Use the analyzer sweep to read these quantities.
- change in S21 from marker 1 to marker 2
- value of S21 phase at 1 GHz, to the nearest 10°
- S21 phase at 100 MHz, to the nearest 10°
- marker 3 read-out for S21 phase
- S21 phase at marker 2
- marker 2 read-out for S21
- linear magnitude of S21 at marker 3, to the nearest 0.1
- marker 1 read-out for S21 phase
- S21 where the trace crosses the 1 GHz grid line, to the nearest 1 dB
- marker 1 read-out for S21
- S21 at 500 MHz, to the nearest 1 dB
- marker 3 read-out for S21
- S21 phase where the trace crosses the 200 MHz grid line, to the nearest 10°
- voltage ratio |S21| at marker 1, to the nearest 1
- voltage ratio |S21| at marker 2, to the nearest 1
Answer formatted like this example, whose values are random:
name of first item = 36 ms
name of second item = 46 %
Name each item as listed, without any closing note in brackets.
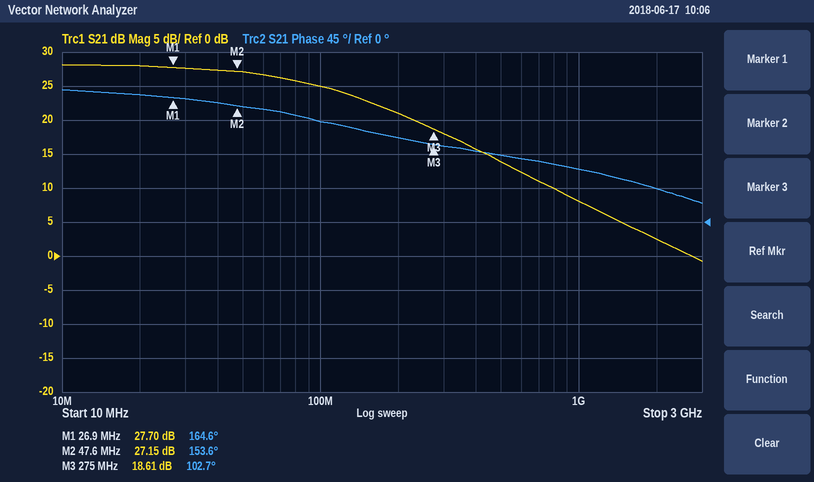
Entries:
change in S21 from marker 1 to marker 2 = -0.55 dB
value of S21 phase at 1 GHz, to the nearest 10° = 70°
S21 phase at 100 MHz, to the nearest 10° = 130°
marker 3 read-out for S21 phase = 102.7°
S21 phase at marker 2 = 153.6°
marker 2 read-out for S21 = 27.15 dB
linear magnitude of S21 at marker 3, to the nearest 0.1 = 8.5
marker 1 read-out for S21 phase = 164.6°
S21 where the trace crosses the 1 GHz grid line, to the nearest 1 dB = 8 dB
marker 1 read-out for S21 = 27.70 dB
S21 at 500 MHz, to the nearest 1 dB = 14 dB
marker 3 read-out for S21 = 18.61 dB
S21 phase where the trace crosses the 200 MHz grid line, to the nearest 10° = 110°
voltage ratio |S21| at marker 1, to the nearest 1 = 24
voltage ratio |S21| at marker 2, to the nearest 1 = 23
